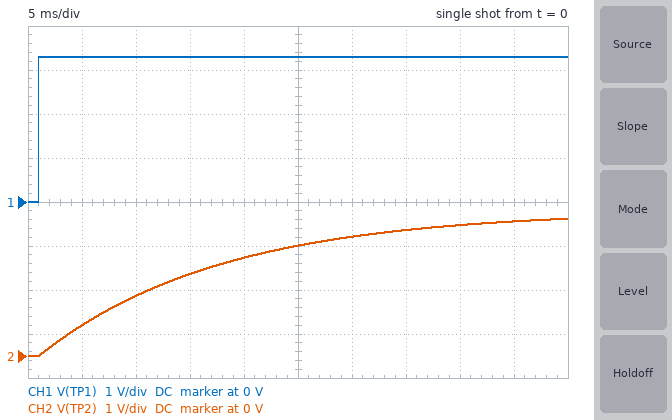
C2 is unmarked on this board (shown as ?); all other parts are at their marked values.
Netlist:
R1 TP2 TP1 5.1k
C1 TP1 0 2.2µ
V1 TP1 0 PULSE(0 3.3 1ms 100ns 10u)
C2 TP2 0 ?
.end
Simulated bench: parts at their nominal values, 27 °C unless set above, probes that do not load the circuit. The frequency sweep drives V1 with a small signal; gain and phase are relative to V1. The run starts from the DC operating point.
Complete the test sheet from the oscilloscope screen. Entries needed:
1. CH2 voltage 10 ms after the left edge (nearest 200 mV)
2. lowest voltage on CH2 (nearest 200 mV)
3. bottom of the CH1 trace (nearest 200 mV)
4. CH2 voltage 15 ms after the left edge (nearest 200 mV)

1.4 V
0 V
0 V
1.8 V
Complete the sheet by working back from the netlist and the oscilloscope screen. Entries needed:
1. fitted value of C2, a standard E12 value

3.3 µF
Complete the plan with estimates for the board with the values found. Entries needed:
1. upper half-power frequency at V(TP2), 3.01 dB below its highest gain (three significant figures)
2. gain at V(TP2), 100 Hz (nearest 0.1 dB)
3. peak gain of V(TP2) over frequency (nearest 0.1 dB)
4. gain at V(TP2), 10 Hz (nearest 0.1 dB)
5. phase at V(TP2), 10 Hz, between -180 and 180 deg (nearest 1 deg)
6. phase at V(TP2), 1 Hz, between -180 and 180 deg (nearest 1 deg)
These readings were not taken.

9.46 Hz
-20.5 dB
0 dB
-3.3 dB
-47 deg
-6 deg
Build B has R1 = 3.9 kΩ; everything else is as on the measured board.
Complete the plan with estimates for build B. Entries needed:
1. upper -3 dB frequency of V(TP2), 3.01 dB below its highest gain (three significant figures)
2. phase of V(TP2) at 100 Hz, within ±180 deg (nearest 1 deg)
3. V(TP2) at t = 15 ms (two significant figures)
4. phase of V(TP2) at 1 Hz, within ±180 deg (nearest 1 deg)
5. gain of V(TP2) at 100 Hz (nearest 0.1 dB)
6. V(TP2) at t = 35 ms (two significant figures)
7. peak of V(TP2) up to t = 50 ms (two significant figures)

12.4 Hz
-83 deg
2.2 V
-5 deg
-18.2 dB
3.1 V
3.2 V
